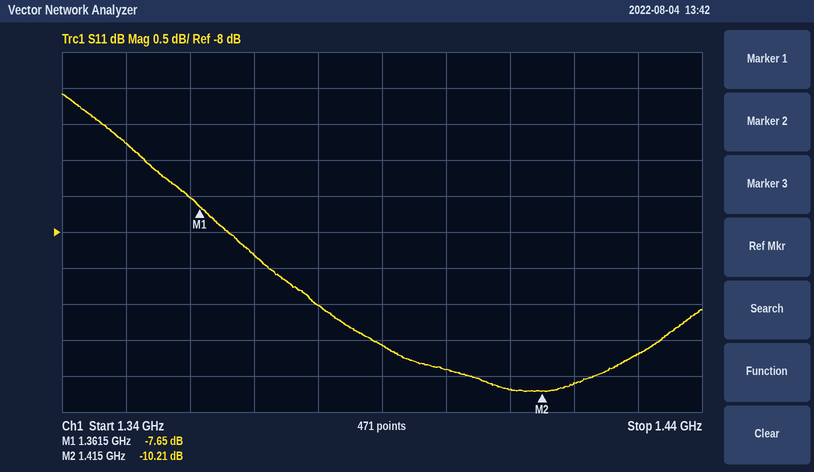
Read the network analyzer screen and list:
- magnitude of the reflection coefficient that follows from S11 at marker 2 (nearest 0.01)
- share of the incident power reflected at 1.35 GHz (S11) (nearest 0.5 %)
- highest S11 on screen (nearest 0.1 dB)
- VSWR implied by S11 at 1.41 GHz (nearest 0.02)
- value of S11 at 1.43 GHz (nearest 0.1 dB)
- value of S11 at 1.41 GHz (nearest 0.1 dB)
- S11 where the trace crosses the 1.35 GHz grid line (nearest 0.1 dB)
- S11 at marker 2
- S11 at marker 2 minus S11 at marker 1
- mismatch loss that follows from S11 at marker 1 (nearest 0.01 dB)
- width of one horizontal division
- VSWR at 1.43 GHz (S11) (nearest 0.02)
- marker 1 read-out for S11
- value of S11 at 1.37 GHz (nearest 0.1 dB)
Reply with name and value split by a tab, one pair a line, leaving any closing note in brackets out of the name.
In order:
magnitude of the reflection coefficient that follows from S11 at marker 2	0.31
share of the incident power reflected at 1.35 GHz (S11)	21.0 %
highest S11 on screen	-6.1 dB
VSWR implied by S11 at 1.41 GHz	1.90
value of S11 at 1.43 GHz	-9.7 dB
value of S11 at 1.41 GHz	-10.2 dB
S11 where the trace crosses the 1.35 GHz grid line	-6.8 dB
S11 at marker 2	-10.21 dB
S11 at marker 2 minus S11 at marker 1	-2.56 dB
mismatch loss that follows from S11 at marker 1	0.82 dB
width of one horizontal division	10 MHz
VSWR at 1.43 GHz (S11)	1.98
marker 1 read-out for S11	-7.65 dB
value of S11 at 1.37 GHz	-8.3 dB
